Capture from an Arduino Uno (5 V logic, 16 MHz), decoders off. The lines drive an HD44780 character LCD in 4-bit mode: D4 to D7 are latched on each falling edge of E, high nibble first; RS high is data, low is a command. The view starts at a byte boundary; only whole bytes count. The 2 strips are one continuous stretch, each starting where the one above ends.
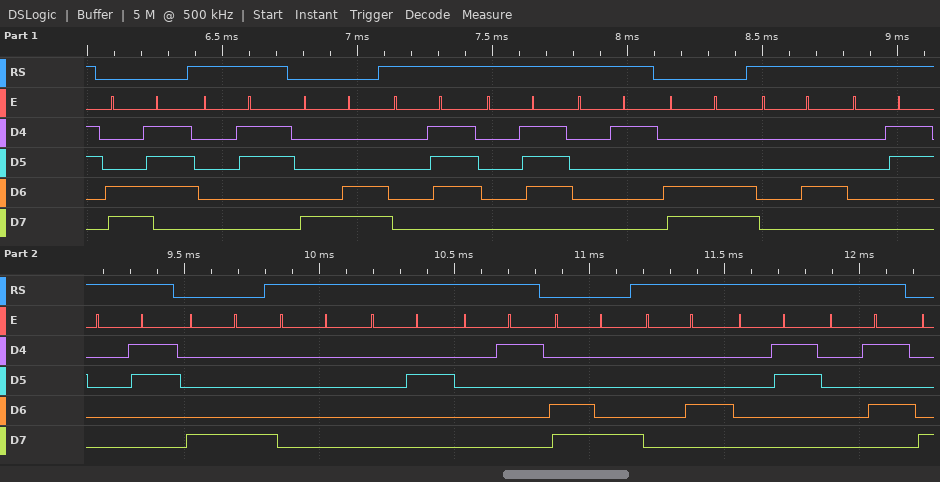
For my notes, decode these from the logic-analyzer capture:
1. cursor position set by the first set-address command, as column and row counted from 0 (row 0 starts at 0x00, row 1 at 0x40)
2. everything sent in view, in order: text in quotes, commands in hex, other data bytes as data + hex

column 7, row 1
0xC7 data 03 0x8C data 07 07 01 0xCC data 04 03 03 0x88 data 00 02 01 0xC8 data 04 03 05
